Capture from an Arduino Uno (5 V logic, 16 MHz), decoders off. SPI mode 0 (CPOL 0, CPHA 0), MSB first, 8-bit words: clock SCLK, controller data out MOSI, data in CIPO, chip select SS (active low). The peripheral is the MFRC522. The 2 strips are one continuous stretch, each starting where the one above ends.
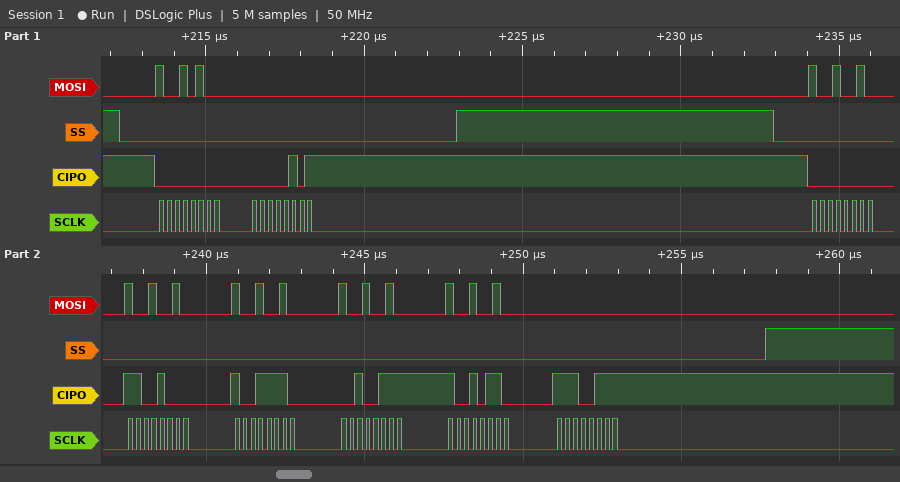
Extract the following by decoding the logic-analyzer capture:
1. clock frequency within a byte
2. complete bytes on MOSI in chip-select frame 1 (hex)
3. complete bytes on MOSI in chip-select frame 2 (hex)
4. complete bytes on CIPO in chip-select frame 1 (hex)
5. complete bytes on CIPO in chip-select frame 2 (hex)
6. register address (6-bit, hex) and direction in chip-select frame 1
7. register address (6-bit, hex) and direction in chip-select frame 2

4 MHz
94 00
92 92 92 92 92 00
00 05
00 C8 9E 27 96 E7
0x0A read
0x09 read
